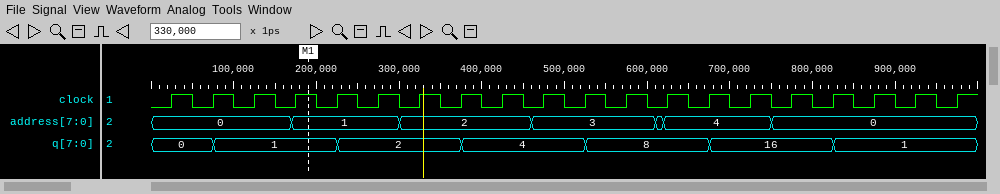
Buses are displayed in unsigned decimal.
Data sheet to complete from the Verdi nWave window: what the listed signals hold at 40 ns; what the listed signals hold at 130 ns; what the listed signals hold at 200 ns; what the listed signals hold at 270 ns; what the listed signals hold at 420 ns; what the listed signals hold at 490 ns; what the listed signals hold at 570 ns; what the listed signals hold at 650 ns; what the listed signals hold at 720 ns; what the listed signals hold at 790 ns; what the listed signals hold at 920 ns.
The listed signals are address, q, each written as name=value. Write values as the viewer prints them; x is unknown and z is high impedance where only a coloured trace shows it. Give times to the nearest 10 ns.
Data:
address=0, q=0
address=0, q=1
address=1, q=1
address=1, q=2
address=2, q=4
address=3, q=4
address=3, q=8
address=4, q=8
address=4, q=16
address=0, q=16
address=0, q=1
